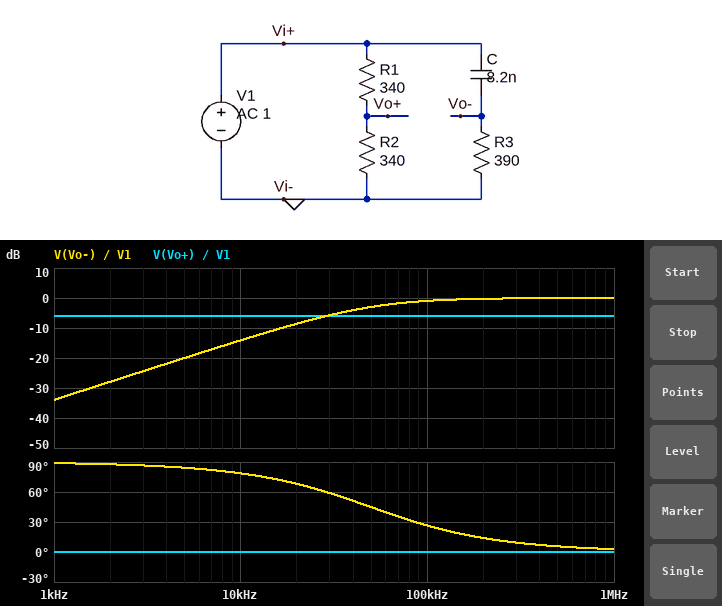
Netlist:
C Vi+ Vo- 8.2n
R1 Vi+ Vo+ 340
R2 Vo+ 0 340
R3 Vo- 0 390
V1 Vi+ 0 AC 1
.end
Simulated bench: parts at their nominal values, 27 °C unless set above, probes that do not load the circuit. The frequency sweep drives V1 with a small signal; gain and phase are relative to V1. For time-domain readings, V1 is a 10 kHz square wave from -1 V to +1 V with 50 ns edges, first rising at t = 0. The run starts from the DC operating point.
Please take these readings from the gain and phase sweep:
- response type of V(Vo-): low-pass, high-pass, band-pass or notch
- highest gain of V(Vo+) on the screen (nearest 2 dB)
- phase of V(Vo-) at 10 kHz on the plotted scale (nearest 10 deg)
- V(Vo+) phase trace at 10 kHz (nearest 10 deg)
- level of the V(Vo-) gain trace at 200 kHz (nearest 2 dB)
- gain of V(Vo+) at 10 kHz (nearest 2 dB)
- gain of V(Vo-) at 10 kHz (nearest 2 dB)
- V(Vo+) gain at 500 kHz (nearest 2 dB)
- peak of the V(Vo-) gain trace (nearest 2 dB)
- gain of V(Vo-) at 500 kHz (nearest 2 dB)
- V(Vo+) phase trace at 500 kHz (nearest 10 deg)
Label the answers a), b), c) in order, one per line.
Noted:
a) high-pass
b) -6 dB
c) 80 deg
d) 0 deg
e) 0 dB
f) -6 dB
g) -14 dB
h) -6 dB
i) 0 dB
j) 0 dB
k) 0 deg
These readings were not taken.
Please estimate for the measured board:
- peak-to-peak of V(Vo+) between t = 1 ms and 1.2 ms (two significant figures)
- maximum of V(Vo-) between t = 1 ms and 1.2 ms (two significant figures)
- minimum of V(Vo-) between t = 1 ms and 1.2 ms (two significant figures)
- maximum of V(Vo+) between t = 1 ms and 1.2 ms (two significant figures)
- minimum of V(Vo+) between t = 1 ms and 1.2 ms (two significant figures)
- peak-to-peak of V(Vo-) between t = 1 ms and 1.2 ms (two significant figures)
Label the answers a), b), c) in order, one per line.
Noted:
a) 1.0 V
b) 2.0 V
c) -2.0 V
d) 500 mV
e) -500 mV
f) 4.0 V
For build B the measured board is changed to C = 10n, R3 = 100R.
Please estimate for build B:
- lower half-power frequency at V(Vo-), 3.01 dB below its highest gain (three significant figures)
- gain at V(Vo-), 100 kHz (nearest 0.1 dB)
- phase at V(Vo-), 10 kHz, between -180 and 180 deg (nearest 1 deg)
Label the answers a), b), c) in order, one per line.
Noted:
a) 159 kHz
b) -5.5 dB
c) 86 deg
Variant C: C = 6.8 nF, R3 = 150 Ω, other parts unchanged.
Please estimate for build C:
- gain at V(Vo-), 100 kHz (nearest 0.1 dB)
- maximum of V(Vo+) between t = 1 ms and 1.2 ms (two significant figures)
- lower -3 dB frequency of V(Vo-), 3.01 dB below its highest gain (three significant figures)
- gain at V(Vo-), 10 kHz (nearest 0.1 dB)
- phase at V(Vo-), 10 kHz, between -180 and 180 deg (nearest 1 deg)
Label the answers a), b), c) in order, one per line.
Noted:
a) -5.4 dB
b) 500 mV
c) 156 kHz
d) -23.9 dB
e) 86 deg
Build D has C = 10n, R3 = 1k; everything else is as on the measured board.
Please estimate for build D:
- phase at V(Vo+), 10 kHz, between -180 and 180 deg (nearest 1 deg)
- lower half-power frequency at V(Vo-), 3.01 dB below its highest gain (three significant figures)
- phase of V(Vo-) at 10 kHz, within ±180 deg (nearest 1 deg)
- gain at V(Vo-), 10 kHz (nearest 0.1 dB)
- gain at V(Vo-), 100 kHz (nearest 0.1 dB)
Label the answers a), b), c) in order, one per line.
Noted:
a) 0 deg
b) 15.9 kHz
c) 58 deg
d) -5.5 dB
e) -0.1 dB
